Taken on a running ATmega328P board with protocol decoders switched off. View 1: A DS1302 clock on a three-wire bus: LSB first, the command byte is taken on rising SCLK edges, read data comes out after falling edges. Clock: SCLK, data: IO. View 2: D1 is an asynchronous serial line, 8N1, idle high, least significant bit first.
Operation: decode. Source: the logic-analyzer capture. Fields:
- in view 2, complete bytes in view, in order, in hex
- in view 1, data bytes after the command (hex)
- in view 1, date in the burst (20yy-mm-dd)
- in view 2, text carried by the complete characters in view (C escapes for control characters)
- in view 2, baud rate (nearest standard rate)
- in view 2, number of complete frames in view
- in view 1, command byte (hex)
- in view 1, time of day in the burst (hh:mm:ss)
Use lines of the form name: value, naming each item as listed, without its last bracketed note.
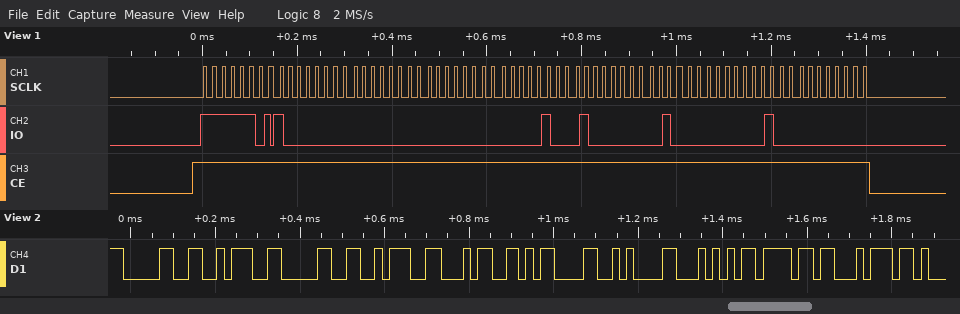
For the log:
in view 2, complete bytes in view, in order, in hex: 0x30 0x3A 0x30 0x3A 0x34 0x0D 0x0A 0x54 0x6F 0x74
in view 1, data bytes after the command: 01 00 00 20 02 04 20 00
in view 1, date in the burst: 2020-02-20
in view 2, text carried by the complete characters in view: "0:0:4\r\nTot"
in view 2, baud rate: 57600 baud
in view 2, number of complete frames in view: 10
in view 1, command byte: 0xBF
in view 1, time of day in the burst: 00:00:01
